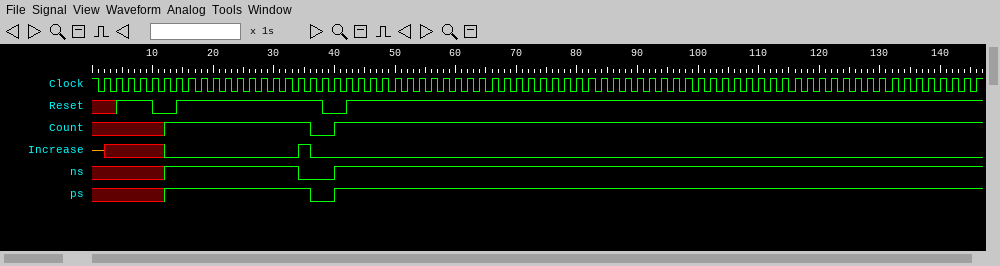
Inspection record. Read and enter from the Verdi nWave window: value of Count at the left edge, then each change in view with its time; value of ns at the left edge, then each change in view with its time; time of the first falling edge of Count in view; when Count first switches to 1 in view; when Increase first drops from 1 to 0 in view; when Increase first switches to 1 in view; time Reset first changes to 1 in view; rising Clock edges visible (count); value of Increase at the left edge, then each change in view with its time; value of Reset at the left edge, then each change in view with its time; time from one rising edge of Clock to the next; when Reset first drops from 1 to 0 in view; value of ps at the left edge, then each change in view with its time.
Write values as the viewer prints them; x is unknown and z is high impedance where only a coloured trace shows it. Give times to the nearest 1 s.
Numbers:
x, 1 at 12 s, 0 at 36 s, 1 at 40 s
x, 1 at 12 s, 0 at 34 s, 1 at 40 s
36 s
12 s
36 s
34 s
4 s
73
z, x at 2 s, 0 at 12 s, 1 at 34 s, 0 at 36 s
x, 1 at 4 s, 0 at 10 s, 1 at 14 s, 0 at 38 s, 1 at 42 s
2 s
10 s
x, 1 at 12 s, 0 at 36 s, 1 at 40 s
